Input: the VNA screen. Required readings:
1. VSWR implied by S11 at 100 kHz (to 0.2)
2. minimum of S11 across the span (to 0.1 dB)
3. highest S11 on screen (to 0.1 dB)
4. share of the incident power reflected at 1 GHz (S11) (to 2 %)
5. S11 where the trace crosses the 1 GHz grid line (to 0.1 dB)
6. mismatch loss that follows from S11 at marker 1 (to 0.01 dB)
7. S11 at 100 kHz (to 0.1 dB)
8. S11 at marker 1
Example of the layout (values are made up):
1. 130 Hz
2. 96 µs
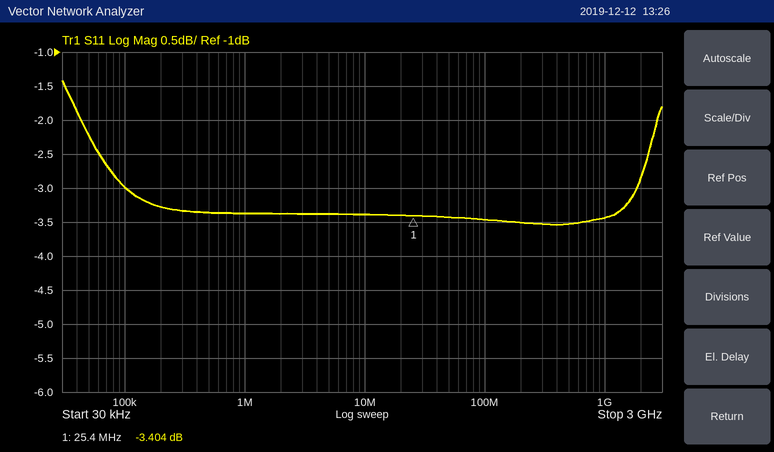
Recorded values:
1. 5.8
2. -3.5 dB
3. -1.4 dB
4. 46 %
5. -3.4 dB
6. 2.65 dB
7. -3.0 dB
8. -3.404 dB
